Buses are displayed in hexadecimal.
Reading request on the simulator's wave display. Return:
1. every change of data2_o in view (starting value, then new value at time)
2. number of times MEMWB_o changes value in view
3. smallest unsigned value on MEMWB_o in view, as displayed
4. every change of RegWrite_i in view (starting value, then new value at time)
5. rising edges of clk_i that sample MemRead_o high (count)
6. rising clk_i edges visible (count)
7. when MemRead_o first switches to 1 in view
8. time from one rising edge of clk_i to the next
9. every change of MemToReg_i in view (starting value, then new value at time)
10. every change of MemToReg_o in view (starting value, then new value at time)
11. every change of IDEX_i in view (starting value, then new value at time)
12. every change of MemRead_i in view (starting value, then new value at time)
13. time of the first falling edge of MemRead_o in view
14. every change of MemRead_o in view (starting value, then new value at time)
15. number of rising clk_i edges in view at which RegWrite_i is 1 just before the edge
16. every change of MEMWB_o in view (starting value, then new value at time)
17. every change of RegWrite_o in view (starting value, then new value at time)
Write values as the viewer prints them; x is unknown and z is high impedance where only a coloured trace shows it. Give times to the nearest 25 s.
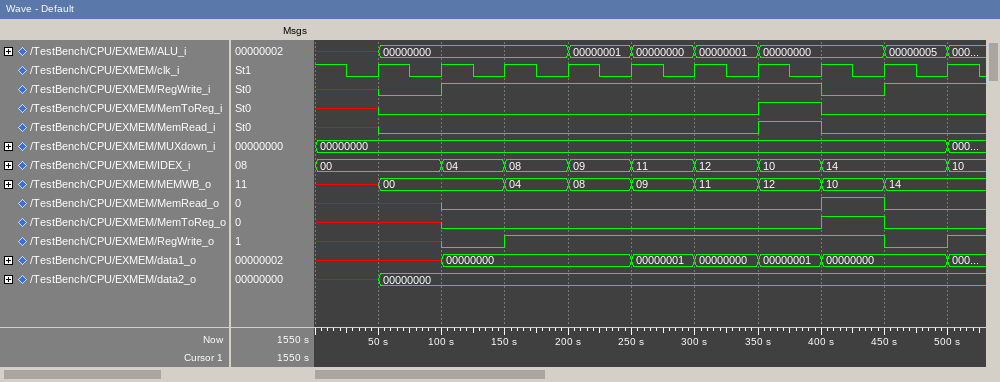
x, 00000000 at 50 s
8
00
x, 0 at 50 s, 1 at 100 s, 0 at 400 s, 1 at 450 s
1
10
400 s
50 s
x, 0 at 50 s, 1 at 350 s, 0 at 400 s
x, 0 at 100 s, 1 at 400 s, 0 at 450 s
00, 04 at 100 s, 08 at 150 s, 09 at 200 s, 11 at 250 s, 12 at 300 s, 10 at 350 s, 14 at 400 s, 10 at 500 s
x, 0 at 50 s, 1 at 350 s, 0 at 400 s
450 s
x, 0 at 100 s, 1 at 400 s, 0 at 450 s
7
x, 00 at 50 s, 04 at 150 s, 08 at 200 s, 09 at 250 s, 11 at 300 s, 12 at 350 s, 10 at 400 s, 14 at 450 s
x, 0 at 100 s, 1 at 150 s, 0 at 450 s, 1 at 500 s
